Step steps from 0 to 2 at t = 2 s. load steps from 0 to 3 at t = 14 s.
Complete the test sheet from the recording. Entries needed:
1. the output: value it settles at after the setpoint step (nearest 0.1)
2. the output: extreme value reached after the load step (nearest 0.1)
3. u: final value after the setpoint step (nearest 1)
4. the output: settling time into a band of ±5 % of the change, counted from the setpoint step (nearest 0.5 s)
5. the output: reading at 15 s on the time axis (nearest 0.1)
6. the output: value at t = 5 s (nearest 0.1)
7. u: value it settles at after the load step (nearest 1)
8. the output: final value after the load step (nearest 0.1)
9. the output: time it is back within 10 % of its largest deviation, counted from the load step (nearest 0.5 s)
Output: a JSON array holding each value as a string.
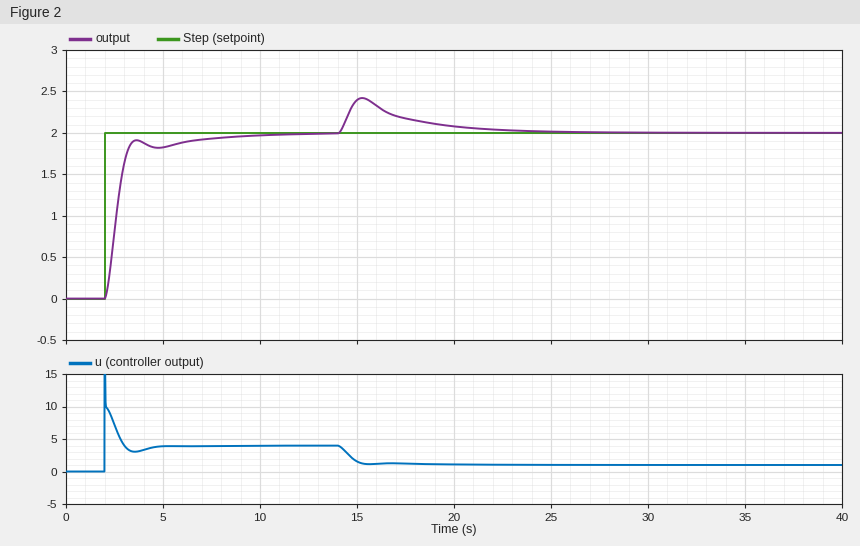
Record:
["2.0", "2.4", "4", "4.5 s", "2.4", "1.8", "1", "2.0", "8.0 s"]
